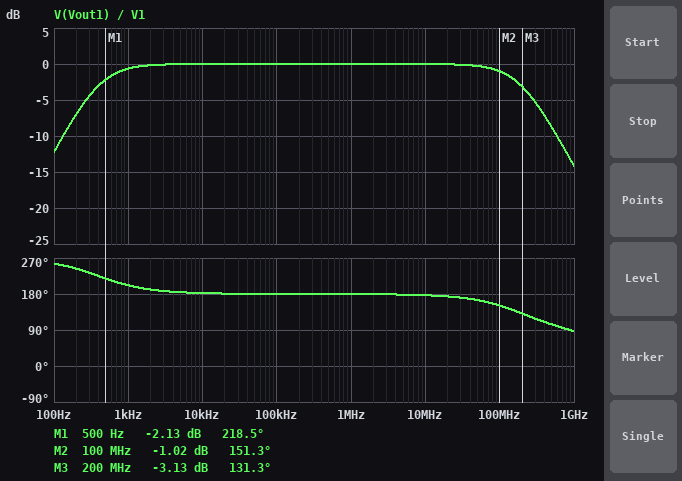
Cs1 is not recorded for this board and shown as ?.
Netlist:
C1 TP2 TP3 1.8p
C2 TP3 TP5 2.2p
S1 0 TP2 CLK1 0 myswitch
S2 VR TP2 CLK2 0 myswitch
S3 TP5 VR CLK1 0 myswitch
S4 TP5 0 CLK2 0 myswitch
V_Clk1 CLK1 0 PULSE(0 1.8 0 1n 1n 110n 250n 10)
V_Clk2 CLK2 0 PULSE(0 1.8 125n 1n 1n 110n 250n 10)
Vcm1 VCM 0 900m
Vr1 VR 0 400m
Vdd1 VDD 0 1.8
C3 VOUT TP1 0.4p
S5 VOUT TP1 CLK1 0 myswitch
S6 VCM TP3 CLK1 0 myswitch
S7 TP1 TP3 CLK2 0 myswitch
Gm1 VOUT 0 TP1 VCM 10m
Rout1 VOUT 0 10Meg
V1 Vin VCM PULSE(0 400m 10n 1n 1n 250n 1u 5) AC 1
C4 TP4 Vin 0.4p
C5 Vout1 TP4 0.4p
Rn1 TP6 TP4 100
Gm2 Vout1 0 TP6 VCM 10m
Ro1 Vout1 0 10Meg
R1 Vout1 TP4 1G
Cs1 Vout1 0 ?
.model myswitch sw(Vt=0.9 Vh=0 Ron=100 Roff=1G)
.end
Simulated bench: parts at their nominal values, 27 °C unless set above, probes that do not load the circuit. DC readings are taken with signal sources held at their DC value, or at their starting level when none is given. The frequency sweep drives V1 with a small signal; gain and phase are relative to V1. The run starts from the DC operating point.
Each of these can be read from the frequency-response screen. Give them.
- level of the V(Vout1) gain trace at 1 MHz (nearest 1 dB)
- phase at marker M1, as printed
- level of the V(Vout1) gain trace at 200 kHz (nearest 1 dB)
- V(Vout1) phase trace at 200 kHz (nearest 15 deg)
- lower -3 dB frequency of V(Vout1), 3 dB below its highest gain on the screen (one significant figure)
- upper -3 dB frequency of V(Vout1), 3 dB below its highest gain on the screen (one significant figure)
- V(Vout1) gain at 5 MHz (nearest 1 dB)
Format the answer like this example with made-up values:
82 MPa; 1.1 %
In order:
0 dB; 218.5 deg; 0 dB; 180 deg; 400 Hz; 200 MHz; 0 dB
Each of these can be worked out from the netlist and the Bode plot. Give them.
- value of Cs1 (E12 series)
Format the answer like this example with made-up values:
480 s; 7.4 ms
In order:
3.9 pF
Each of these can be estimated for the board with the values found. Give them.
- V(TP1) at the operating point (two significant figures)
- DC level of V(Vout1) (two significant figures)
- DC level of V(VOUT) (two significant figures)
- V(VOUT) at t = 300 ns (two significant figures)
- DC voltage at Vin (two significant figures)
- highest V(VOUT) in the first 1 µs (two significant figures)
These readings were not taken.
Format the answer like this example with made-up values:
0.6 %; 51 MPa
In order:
900 mV; 900 mV; 900 mV; 900 mV; 900 mV; 1.3 V
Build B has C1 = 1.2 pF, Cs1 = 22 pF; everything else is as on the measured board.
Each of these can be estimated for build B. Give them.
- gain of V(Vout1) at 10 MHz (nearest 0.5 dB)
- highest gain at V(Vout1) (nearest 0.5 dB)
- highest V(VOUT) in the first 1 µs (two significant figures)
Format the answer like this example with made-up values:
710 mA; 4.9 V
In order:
-0.5 dB; 0 dB; 1.9 V
